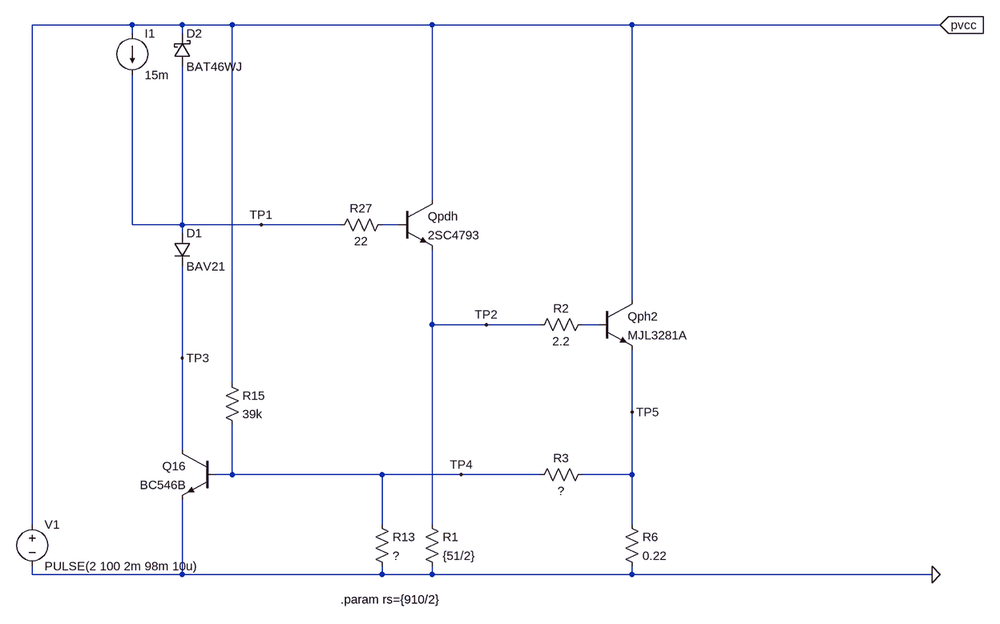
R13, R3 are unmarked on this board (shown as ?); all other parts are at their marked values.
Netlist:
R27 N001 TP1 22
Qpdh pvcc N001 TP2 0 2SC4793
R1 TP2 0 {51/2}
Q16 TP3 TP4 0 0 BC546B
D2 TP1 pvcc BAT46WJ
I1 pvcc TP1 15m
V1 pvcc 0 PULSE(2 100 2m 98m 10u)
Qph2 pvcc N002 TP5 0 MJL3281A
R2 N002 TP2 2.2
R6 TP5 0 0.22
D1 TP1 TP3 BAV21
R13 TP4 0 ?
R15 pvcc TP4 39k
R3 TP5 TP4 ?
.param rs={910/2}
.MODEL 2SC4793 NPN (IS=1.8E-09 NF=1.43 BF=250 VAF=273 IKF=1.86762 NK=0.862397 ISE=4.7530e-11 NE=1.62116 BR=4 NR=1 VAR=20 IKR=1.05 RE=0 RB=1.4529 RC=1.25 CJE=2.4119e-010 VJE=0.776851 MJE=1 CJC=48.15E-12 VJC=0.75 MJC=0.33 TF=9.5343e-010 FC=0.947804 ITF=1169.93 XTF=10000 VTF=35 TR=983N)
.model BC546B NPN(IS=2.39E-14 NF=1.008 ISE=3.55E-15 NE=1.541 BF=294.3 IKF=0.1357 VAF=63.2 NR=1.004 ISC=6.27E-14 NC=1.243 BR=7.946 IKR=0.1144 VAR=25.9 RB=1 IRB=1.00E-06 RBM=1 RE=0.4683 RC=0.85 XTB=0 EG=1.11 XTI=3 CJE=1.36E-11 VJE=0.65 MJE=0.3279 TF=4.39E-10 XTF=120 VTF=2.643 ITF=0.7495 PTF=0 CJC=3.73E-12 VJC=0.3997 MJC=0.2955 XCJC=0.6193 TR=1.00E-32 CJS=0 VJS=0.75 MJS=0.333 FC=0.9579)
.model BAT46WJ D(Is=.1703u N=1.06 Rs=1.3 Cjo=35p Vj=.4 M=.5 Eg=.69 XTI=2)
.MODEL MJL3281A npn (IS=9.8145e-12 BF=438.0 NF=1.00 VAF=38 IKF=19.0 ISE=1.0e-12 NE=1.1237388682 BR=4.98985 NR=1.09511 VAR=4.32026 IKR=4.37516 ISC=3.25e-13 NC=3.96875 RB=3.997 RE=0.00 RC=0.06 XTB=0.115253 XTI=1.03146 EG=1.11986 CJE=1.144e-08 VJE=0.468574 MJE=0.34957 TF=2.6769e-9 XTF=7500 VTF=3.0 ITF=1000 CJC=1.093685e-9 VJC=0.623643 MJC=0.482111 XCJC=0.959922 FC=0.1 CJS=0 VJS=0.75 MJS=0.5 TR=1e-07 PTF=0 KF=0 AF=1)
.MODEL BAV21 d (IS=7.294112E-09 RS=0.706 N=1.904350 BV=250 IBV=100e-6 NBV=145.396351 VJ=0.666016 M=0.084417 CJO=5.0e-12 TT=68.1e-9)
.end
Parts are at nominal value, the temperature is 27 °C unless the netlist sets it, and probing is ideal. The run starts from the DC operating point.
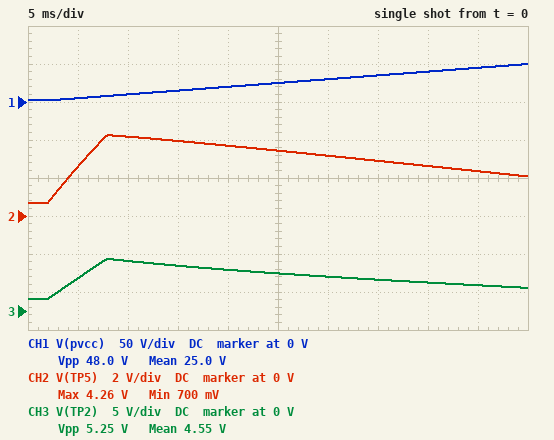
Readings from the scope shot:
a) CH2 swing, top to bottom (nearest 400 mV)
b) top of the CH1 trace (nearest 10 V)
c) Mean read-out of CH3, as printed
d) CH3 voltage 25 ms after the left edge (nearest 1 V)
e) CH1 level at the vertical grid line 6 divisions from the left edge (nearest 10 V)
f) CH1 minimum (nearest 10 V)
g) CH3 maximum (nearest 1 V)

3.6 V
50 V
4.55 V
5 V
30 V
0 V
7 V
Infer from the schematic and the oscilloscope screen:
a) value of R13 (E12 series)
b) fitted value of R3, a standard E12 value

390 Ω
2.2 kΩ
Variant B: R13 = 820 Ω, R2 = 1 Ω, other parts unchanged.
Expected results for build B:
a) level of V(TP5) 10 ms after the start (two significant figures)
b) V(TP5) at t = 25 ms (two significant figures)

2.2 V
1.4 V
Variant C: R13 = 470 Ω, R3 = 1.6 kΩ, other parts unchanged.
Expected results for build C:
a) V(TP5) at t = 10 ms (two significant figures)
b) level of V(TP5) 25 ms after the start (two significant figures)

2.8 V
2.2 V
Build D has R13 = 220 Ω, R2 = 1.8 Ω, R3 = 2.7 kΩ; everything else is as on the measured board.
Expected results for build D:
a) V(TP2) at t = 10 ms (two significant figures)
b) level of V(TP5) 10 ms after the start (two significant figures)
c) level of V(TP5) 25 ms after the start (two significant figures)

8.7 V
5.5 V
7.1 V
